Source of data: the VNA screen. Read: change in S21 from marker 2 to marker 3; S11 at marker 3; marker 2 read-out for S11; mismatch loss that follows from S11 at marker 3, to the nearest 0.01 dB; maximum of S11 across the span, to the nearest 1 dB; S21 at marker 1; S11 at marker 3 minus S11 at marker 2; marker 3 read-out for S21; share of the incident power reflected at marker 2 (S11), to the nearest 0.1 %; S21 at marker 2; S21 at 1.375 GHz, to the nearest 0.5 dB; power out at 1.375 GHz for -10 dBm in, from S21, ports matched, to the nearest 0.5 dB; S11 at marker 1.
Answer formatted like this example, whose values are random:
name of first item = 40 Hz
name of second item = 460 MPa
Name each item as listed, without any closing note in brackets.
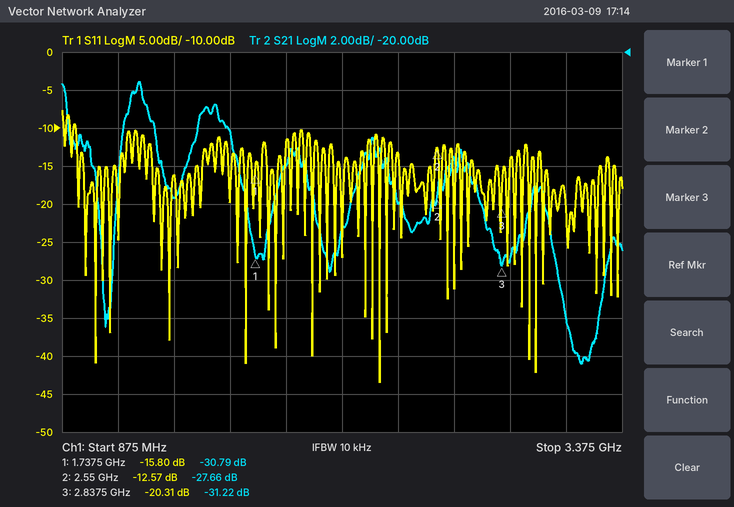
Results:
change in S21 from marker 2 to marker 3 = -3.56 dB
S11 at marker 3 = -20.31 dB
marker 2 read-out for S11 = -12.57 dB
mismatch loss that follows from S11 at marker 3, to the nearest 0.01 dB = 0.04 dB
maximum of S11 across the span, to the nearest 1 dB = -8 dB
S21 at marker 1 = -30.79 dB
S11 at marker 3 minus S11 at marker 2 = -7.74 dB
marker 3 read-out for S21 = -31.22 dB
share of the incident power reflected at marker 2 (S11), to the nearest 0.1 % = 5.5 %
S21 at marker 2 = -27.66 dB
S21 at 1.375 GHz, to the nearest 0.5 dB = -27.5 dB
power out at 1.375 GHz for -10 dBm in, from S21, ports matched, to the nearest 0.5 dB = -37.5 dBm
S11 at marker 1 = -15.80 dB
